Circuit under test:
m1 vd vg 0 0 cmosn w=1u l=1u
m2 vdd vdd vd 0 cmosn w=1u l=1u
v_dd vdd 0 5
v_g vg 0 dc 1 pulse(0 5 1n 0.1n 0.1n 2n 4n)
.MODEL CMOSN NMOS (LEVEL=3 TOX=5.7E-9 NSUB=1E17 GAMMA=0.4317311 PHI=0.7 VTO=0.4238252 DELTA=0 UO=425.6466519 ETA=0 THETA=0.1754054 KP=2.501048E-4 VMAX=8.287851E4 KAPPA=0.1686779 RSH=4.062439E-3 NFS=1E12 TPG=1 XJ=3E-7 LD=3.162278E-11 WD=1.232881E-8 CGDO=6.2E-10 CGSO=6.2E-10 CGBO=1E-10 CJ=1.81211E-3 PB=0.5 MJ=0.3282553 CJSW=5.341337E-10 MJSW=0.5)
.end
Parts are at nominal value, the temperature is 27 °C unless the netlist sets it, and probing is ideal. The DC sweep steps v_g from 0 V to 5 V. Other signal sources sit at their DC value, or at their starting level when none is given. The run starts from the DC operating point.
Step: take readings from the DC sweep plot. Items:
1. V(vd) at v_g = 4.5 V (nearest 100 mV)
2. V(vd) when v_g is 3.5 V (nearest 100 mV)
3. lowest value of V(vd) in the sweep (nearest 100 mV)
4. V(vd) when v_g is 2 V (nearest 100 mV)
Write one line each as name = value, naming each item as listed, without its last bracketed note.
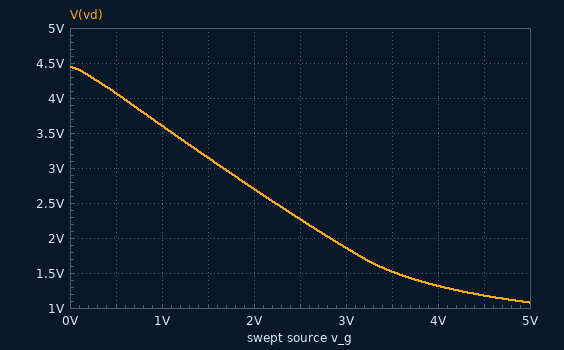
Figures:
V(vd) at v_g = 4.5 V = 1.2 V
V(vd) when v_g is 3.5 V = 1.5 V
lowest value of V(vd) in the sweep = 1.1 V
V(vd) when v_g is 2 V = 2.7 V
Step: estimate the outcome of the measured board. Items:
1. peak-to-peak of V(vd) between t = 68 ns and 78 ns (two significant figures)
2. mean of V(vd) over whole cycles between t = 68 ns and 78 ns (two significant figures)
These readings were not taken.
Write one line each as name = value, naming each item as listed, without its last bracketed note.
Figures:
peak-to-peak of V(vd) between t = 68 ns and 78 ns = 3.3 V
mean of V(vd) over whole cycles between t = 68 ns and 78 ns = 2.5 V
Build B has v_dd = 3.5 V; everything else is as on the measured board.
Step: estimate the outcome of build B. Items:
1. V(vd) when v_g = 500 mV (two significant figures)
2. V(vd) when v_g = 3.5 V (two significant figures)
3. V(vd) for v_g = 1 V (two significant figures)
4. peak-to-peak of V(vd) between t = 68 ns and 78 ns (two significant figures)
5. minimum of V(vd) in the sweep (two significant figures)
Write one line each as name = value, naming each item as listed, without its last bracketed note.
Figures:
V(vd) when v_g = 500 mV = 2.7 V
V(vd) when v_g = 3.5 V = 740 mV
V(vd) for v_g = 1 V = 2.2 V
peak-to-peak of V(vd) between t = 68 ns and 78 ns = 2.5 V
minimum of V(vd) in the sweep = 570 mV
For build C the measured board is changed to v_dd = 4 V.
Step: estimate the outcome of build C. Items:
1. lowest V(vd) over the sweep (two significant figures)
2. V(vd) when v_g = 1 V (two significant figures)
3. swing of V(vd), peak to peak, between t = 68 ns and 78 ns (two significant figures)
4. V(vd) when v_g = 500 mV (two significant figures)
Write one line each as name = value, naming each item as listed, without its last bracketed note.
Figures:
lowest V(vd) over the sweep = 720 mV
V(vd) when v_g = 1 V = 2.7 V
swing of V(vd), peak to peak, between t = 68 ns and 78 ns = 2.8 V
V(vd) when v_g = 500 mV = 3.1 V
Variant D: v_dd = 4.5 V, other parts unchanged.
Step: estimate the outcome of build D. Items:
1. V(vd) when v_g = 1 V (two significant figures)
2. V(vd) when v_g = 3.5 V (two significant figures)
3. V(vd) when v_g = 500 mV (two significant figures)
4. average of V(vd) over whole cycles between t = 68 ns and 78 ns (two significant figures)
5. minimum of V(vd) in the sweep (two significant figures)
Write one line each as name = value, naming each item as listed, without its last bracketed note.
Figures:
V(vd) when v_g = 1 V = 3.1 V
V(vd) when v_g = 3.5 V = 1.2 V
V(vd) when v_g = 500 mV = 3.6 V
average of V(vd) over whole cycles between t = 68 ns and 78 ns = 2.2 V
minimum of V(vd) in the sweep = 890 mV
